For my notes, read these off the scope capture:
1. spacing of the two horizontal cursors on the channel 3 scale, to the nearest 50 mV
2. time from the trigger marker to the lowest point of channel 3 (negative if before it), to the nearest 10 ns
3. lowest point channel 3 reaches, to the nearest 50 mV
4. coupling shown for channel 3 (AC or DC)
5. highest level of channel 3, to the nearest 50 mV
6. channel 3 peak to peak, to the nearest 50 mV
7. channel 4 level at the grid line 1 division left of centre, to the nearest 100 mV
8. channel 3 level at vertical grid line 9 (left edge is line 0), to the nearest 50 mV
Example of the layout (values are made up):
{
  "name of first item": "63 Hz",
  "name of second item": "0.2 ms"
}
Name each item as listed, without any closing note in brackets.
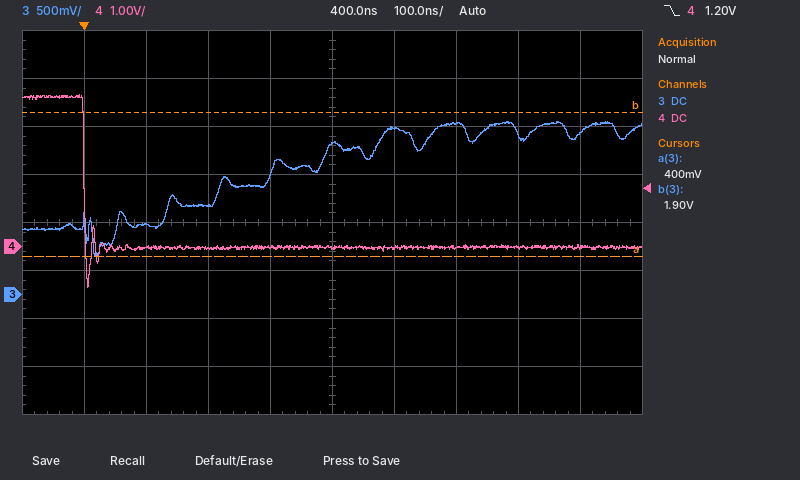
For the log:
{
  "spacing of the two horizontal cursors on the channel 3 scale, to the nearest 50 mV": "1.50 V",
  "time from the trigger marker to the lowest point of channel 3 (negative if before it), to the nearest 10 ns": "+20 ns",
  "lowest point channel 3 reaches, to the nearest 50 mV": "400 mV",
  "coupling shown for channel 3": "DC",
  "highest level of channel 3, to the nearest 50 mV": "1.80 V",
  "channel 3 peak to peak, to the nearest 50 mV": "1.40 V",
  "channel 4 level at the grid line 1 division left of centre, to the nearest 100 mV": "0.0 V",
  "channel 3 level at vertical grid line 9 (left edge is line 0), to the nearest 50 mV": "1.70 V"
}
